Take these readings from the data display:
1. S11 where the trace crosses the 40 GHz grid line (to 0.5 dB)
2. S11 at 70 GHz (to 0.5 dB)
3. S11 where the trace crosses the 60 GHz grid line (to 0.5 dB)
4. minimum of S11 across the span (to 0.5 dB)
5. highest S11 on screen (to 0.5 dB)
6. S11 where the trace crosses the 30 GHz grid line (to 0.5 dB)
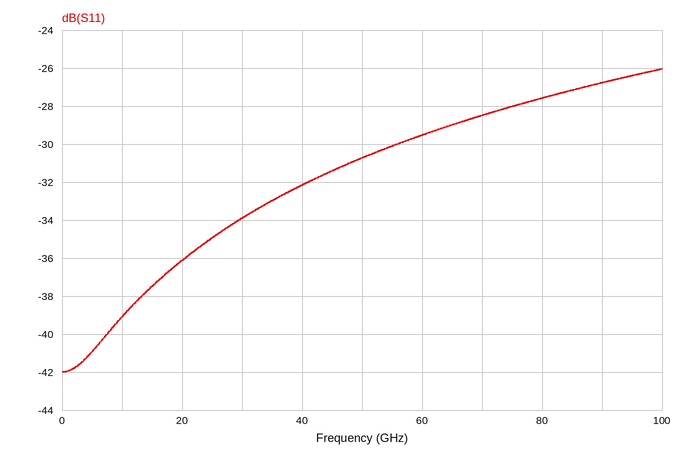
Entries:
-32.0 dB
-28.5 dB
-29.5 dB
-42.0 dB
-26.0 dB
-34.0 dB
